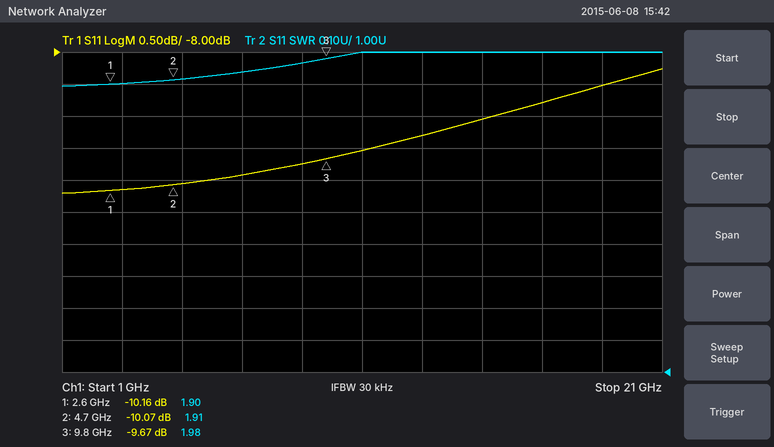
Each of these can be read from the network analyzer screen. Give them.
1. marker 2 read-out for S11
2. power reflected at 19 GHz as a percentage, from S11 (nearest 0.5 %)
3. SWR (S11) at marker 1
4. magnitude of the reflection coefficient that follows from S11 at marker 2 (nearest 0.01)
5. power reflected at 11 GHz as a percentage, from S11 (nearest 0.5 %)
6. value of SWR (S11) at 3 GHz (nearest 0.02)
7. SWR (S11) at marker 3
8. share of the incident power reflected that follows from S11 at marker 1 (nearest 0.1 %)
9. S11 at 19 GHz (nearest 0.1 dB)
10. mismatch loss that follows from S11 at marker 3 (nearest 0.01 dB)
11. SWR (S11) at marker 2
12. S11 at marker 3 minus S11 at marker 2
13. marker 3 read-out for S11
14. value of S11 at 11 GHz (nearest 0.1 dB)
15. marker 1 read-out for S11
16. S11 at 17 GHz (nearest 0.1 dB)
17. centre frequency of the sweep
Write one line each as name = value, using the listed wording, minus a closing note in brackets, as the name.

marker 2 read-out for S11 = -10.07 dB
power reflected at 19 GHz as a percentage, from S11 = 14.0 %
SWR (S11) at marker 1 = 1.90
magnitude of the reflection coefficient that follows from S11 at marker 2 = 0.31
power reflected at 11 GHz as a percentage, from S11 = 11.0 %
value of SWR (S11) at 3 GHz = 1.90
SWR (S11) at marker 3 = 1.98
share of the incident power reflected that follows from S11 at marker 1 = 9.6 %
S11 at 19 GHz = -8.5 dB
mismatch loss that follows from S11 at marker 3 = 0.50 dB
SWR (S11) at marker 2 = 1.91
S11 at marker 3 minus S11 at marker 2 = 0.40 dB
marker 3 read-out for S11 = -9.67 dB
value of S11 at 11 GHz = -9.5 dB
marker 1 read-out for S11 = -10.16 dB
S11 at 17 GHz = -8.8 dB
centre frequency of the sweep = 11 GHz
